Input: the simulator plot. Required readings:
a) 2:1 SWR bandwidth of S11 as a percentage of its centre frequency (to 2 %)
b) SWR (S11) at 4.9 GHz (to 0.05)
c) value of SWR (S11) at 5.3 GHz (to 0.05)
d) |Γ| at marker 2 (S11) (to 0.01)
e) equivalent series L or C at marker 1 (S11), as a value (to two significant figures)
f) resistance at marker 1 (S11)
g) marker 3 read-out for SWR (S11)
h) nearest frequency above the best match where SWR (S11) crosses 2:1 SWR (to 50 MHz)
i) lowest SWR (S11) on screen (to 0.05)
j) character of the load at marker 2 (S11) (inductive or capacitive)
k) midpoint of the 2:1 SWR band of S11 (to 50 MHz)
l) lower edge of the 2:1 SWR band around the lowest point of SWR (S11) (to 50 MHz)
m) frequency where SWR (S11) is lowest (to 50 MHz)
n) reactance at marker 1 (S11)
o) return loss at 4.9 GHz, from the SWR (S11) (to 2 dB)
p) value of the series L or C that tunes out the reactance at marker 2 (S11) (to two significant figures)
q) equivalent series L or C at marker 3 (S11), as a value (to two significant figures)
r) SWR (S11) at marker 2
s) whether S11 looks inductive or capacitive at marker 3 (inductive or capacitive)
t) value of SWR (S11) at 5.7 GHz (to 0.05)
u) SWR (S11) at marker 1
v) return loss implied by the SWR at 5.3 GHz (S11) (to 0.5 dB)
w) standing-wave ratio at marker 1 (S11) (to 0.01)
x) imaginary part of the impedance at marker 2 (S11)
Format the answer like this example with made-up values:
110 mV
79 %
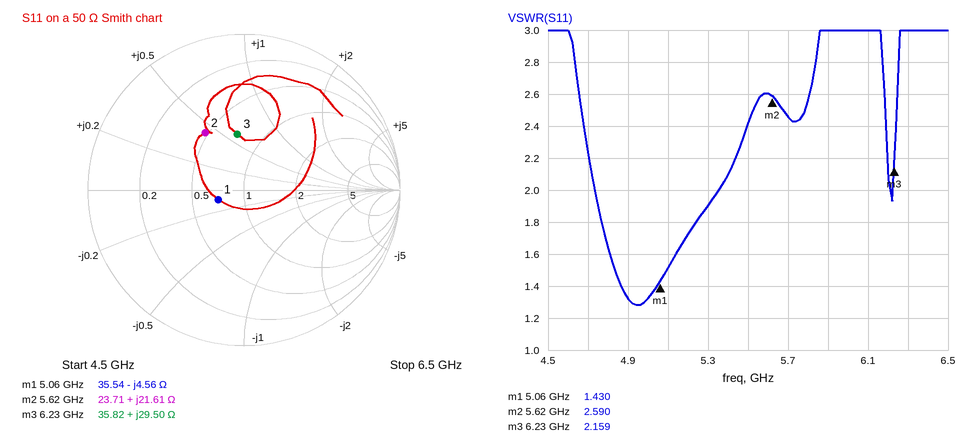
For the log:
12 %
1.30
1.90
0.44
6.9 pF
35.54 Ω
2.159
5.35 GHz
1.30
inductive
5.05 GHz
4.75 GHz
4.95 GHz
-4.56 Ω
18 dB
1.3 pF
750 pH
2.590
inductive
2.45
1.430
10.0 dB
1.43
+21.61 Ω
